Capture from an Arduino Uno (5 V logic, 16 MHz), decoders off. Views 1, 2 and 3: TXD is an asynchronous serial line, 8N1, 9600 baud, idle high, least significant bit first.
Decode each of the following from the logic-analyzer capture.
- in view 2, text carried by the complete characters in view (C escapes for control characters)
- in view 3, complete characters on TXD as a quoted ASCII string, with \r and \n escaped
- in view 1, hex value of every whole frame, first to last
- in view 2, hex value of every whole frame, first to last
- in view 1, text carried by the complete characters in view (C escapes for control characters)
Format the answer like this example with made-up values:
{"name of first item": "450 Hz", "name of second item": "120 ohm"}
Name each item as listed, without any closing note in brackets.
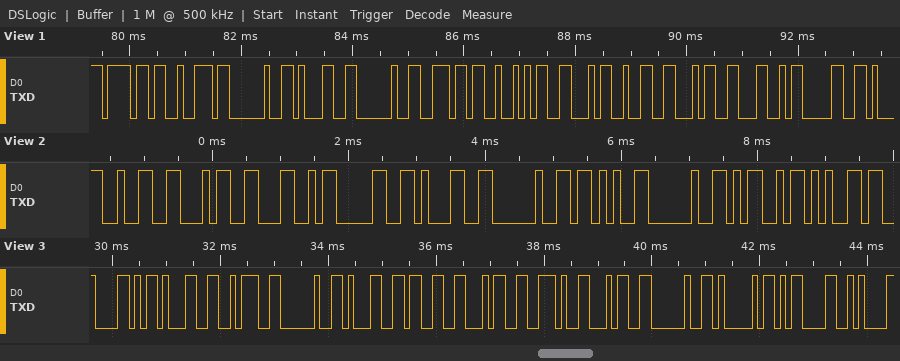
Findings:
{"in view 2, text carried by the complete characters in view": "\"24L01 + Me\"", "in view 3, complete characters on TXD as a quoted ASCII string, with \\r and \\n escaped": "\"X1: 134.4 A\\r\\n\"", "in view 1, hex value of every whole frame, first to last": "6F 72 20 31 20 6E 52 46 32 34 4C 30", "in view 2, hex value of every whole frame, first to last": "32 34 4C 30 31 20 2B 20 4D 65", "in view 1, text carried by the complete characters in view": "\"or 1 nRF24L0\""}
